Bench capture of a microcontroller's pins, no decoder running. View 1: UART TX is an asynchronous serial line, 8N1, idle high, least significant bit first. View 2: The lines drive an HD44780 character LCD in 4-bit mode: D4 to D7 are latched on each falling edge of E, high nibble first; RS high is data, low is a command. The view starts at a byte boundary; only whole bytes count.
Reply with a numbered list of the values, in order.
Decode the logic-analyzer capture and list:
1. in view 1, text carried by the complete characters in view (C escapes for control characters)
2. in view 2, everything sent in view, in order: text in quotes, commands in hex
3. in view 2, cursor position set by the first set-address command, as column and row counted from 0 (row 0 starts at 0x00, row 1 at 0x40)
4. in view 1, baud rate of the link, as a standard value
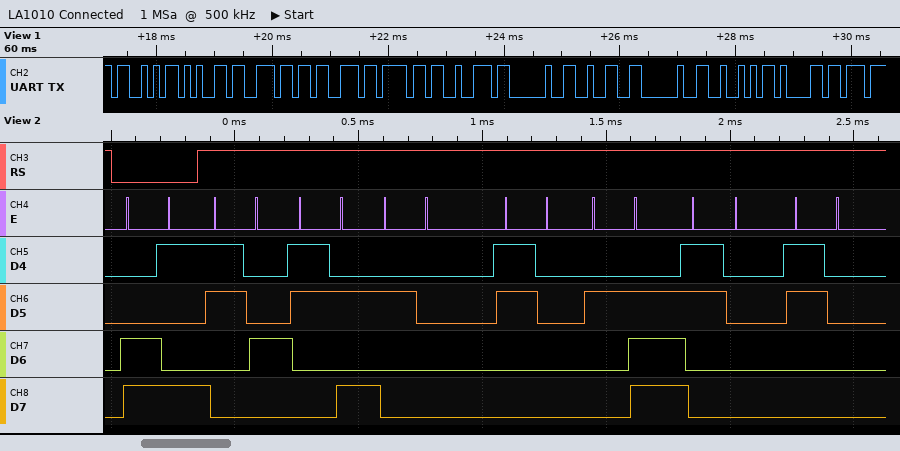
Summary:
1. "Sensor 2 Ra"
2. 0xC9 "4: 0.00"
3. column 9, row 1
4. 9600 baud
